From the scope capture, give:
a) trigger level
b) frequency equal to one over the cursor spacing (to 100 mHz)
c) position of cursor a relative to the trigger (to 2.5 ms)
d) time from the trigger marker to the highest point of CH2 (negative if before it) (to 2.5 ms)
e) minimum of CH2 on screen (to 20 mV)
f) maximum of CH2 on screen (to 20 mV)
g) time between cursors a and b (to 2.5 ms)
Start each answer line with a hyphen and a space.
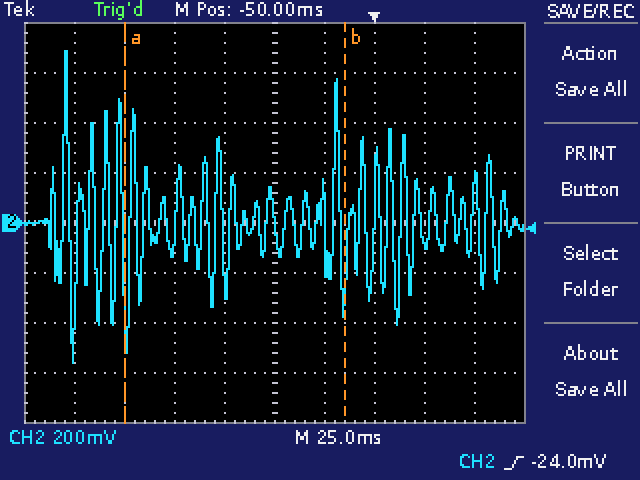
- -24.0 mV
- 9.1 Hz
- -125.0 ms
- -155.0 ms
- -560 mV
- 680 mV
- 110.0 ms
